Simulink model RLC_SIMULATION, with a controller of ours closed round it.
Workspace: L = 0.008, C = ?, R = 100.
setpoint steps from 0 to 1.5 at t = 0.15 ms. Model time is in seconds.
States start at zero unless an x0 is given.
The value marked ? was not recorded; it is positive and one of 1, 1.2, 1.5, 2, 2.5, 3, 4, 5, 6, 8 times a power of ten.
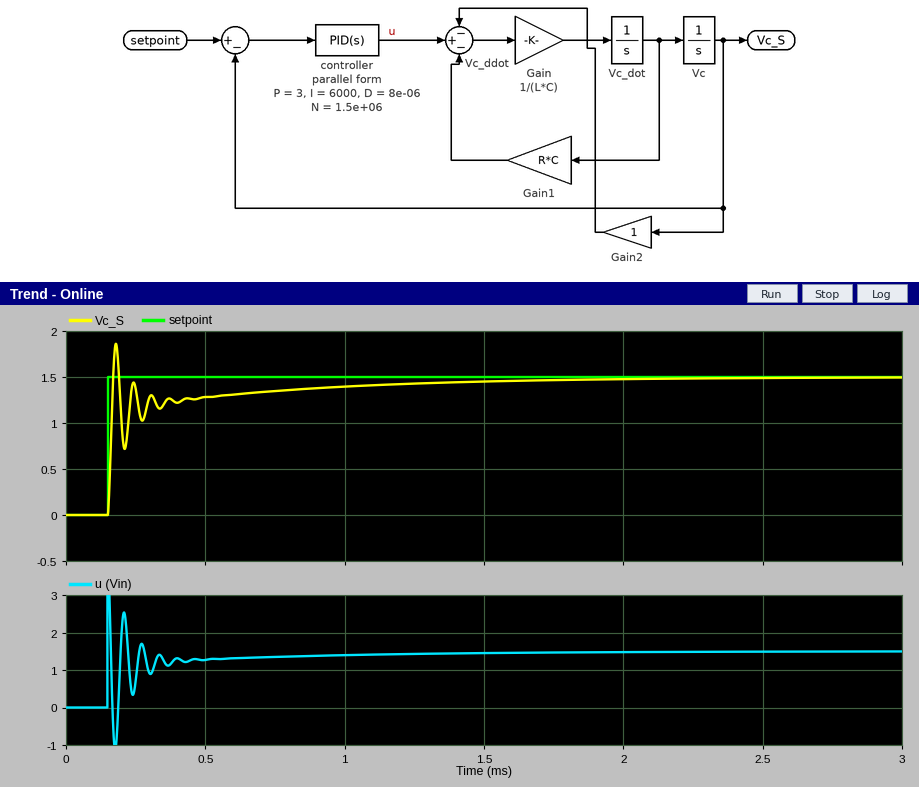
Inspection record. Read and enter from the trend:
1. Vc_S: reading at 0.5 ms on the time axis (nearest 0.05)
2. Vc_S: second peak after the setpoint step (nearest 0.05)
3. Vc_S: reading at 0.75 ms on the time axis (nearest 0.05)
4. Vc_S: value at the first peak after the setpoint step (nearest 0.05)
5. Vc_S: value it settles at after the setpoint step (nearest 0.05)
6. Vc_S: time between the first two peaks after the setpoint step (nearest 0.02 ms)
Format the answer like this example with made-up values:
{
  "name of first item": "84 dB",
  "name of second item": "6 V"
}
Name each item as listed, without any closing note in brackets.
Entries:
{
  "Vc_S: reading at 0.5 ms on the time axis": "1.30",
  "Vc_S: second peak after the setpoint step": "1.45",
  "Vc_S: reading at 0.75 ms on the time axis": "1.35",
  "Vc_S: value at the first peak after the setpoint step": "1.85",
  "Vc_S: value it settles at after the setpoint step": "1.50",
  "Vc_S: time between the first two peaks after the setpoint step": "0.06 ms"
}
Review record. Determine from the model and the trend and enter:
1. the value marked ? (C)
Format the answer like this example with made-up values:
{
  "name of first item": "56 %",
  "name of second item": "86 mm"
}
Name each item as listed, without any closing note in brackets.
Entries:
{
  "the value marked ?": "5e-08"
}
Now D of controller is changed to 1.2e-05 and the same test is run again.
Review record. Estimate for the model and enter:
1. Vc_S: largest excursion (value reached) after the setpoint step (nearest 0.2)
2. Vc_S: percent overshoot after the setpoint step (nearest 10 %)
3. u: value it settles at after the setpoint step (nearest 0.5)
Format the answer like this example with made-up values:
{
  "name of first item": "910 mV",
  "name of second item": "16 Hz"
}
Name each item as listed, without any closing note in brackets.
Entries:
{
  "Vc_S: largest excursion (value reached) after the setpoint step": "1.8",
  "Vc_S: percent overshoot after the setpoint step": "20 %",
  "u: value it settles at after the setpoint step": "1.5"
}
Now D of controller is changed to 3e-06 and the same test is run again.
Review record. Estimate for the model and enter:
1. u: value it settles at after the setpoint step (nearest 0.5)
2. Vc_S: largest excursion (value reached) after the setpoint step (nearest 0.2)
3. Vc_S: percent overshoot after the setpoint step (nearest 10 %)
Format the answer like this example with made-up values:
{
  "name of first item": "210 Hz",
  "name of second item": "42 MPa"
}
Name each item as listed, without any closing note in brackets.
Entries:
{
  "u: value it settles at after the setpoint step": "1.5",
  "Vc_S: largest excursion (value reached) after the setpoint step": "2.0",
  "Vc_S: percent overshoot after the setpoint step": "30 %"
}
